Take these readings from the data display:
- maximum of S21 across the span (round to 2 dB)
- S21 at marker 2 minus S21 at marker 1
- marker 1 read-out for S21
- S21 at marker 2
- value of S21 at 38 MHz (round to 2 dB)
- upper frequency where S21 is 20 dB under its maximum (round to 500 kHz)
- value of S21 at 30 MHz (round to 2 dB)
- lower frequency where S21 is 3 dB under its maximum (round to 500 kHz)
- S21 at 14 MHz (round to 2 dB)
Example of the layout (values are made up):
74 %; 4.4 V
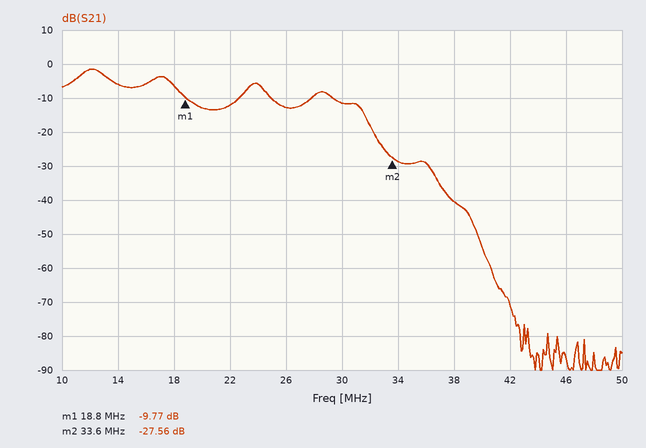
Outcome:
-2 dB; -17.79 dB; -9.77 dB; -27.56 dB; -40 dB; 32.5 MHz; -12 dB; 11.0 MHz; -6 dB
